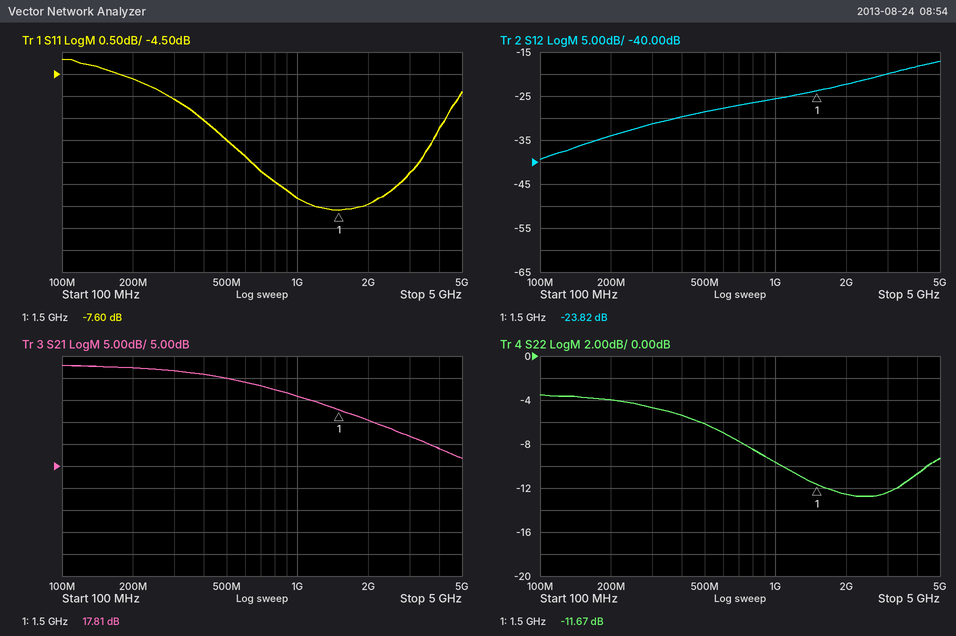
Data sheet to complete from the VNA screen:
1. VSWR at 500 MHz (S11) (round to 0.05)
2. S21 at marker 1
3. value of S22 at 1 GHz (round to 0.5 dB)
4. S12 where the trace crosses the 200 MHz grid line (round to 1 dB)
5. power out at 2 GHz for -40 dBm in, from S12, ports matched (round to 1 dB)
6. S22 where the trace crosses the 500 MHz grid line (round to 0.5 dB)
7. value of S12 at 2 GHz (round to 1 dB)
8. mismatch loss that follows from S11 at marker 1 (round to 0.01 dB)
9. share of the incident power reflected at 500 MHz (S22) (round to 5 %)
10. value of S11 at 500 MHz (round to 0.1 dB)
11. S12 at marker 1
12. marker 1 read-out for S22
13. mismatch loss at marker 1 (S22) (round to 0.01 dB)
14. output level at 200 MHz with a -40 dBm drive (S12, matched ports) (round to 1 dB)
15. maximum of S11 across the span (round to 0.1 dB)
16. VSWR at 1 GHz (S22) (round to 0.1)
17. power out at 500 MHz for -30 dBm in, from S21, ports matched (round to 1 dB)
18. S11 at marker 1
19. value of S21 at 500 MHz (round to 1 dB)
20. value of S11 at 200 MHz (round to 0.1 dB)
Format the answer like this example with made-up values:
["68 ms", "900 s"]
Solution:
["3.00", "17.81 dB", "-9.5 dB", "-34 dB", "-62 dBm", "-6.0 dB", "-22 dB", "0.83 dB", "25 %", "-6.0 dB", "-23.82 dB", "-11.67 dB", "0.31 dB", "-74 dBm", "-4.2 dB", "2.0", "-5 dBm", "-7.60 dB", "25 dB", "-4.6 dB"]
